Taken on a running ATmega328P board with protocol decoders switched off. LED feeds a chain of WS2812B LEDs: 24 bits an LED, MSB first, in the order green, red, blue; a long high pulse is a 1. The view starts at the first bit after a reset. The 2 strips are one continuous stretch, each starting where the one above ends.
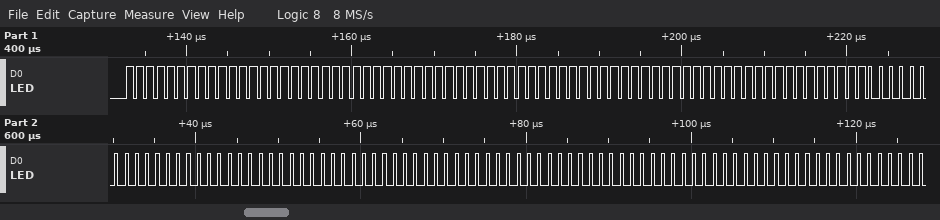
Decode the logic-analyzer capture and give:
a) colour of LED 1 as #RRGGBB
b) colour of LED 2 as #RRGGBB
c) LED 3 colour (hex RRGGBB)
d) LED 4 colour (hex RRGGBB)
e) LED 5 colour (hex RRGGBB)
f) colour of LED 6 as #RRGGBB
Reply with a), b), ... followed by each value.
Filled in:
a) #FFFFFF
b) #FFFFFF
c) #FFFFFF
d) #000000
e) #000000
f) #000000
